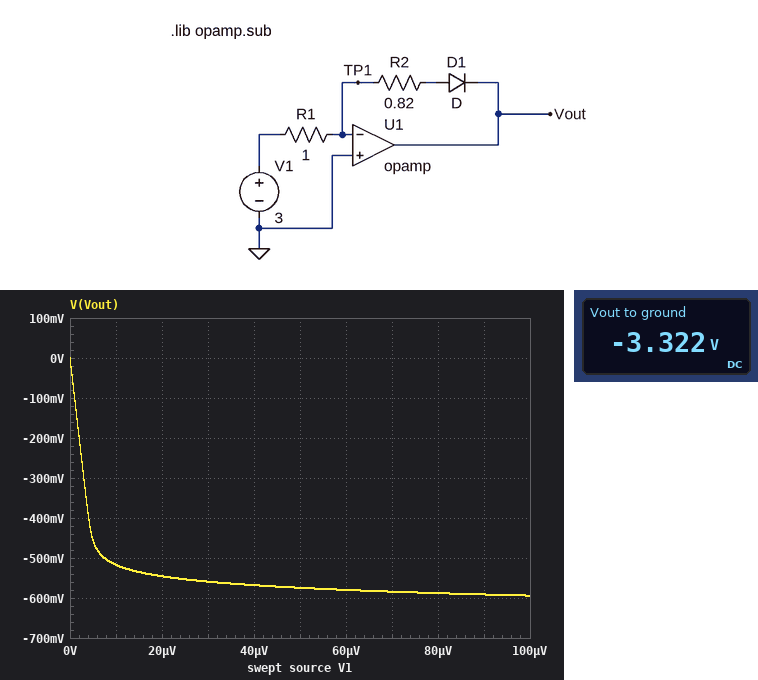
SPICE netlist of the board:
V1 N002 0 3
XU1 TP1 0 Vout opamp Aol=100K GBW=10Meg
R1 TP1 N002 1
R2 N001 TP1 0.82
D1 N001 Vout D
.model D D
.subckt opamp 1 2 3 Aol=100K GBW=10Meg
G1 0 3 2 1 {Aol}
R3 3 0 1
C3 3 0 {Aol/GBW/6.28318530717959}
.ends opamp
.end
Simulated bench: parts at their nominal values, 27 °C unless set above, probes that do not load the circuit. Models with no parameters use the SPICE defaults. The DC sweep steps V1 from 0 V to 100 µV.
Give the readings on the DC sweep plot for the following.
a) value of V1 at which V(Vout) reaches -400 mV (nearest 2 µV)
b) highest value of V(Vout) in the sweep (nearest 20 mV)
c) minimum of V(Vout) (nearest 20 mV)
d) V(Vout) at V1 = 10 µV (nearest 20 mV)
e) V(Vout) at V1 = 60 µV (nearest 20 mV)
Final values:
4 µV
0 V
-600 mV
-520 mV
-580 mV
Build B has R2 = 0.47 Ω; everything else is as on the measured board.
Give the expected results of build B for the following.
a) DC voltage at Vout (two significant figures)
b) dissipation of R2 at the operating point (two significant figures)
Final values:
-2.3 V
4.2 W
